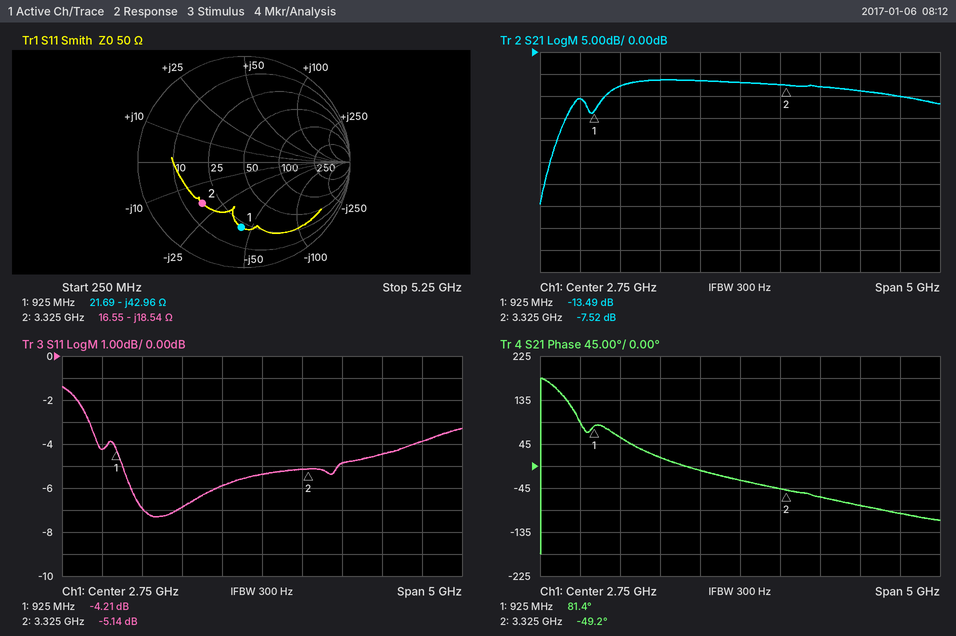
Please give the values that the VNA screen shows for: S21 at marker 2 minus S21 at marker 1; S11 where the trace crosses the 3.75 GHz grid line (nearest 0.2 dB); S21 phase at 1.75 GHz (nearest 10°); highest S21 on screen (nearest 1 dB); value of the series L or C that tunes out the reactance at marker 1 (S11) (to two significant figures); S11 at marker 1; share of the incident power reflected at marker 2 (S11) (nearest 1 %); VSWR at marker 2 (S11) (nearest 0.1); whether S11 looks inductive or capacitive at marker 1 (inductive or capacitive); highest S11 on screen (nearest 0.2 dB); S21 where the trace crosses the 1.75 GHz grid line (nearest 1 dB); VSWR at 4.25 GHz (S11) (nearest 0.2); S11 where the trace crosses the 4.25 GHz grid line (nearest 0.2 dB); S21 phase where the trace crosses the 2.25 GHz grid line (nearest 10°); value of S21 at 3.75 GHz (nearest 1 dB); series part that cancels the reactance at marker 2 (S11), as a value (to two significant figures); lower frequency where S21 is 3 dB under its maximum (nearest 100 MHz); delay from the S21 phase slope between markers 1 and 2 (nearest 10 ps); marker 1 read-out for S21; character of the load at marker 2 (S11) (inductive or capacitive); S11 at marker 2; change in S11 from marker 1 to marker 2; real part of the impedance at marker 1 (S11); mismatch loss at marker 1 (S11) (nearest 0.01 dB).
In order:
5.97 dB
-4.8 dB
20°
-6 dB
7.4 nH
-4.21 dB
31 %
3.5
capacitive
-1.4 dB
-6 dB
4.0
-4.4 dB
-10°
-8 dB
890 pH
1.1 GHz
150 ps
-13.49 dB
capacitive
-5.14 dB
-0.93 dB
21.69 Ω
2.07 dB
